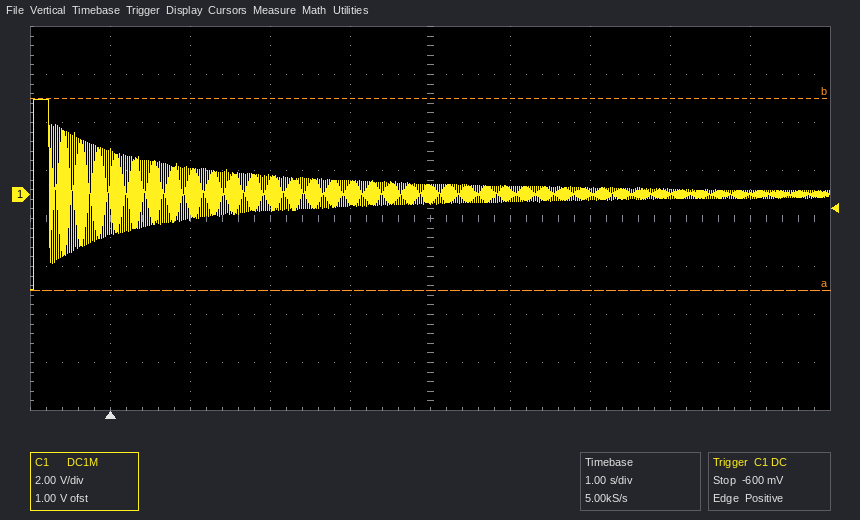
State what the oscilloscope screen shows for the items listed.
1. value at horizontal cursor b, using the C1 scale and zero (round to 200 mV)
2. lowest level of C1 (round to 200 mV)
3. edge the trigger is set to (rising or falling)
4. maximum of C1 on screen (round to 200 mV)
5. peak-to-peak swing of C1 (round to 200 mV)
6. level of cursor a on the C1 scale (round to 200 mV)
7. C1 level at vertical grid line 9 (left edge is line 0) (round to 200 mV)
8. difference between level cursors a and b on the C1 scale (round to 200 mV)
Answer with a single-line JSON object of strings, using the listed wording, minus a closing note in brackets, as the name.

{"value at horizontal cursor b, using the C1 scale and zero": "4.0 V", "lowest level of C1": "-4.0 V", "edge the trigger is set to": "rising", "maximum of C1 on screen": "4.0 V", "peak-to-peak swing of C1": "8.0 V", "level of cursor a on the C1 scale": "-4.0 V", "C1 level at vertical grid line 9 (left edge is line 0)": "0.0 V", "difference between level cursors a and b on the C1 scale": "8.0 V"}
